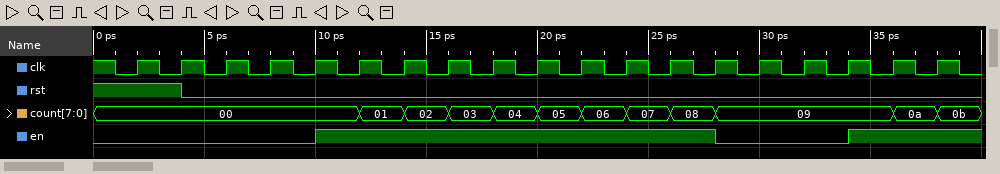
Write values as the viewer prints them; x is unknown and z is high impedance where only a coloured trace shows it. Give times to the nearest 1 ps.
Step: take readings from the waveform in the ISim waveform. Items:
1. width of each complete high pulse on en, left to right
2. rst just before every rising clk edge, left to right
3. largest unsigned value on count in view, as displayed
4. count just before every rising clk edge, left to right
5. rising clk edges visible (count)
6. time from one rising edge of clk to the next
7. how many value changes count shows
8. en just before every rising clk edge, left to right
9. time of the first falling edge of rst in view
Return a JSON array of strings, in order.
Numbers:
["18 ps", "1 1 0 0 0 0 0 0 0 0 0 0 0 0 0 0 0 0 0", "0b", "00, 00, 00, 00, 00, 00, 01, 02, 03, 04, 05, 06, 07, 08, 09, 09, 09, 09, 0a", "19", "2 ps", "11", "0 0 0 0 0 1 1 1 1 1 1 1 1 1 0 0 0 1 1", "4 ps"]
